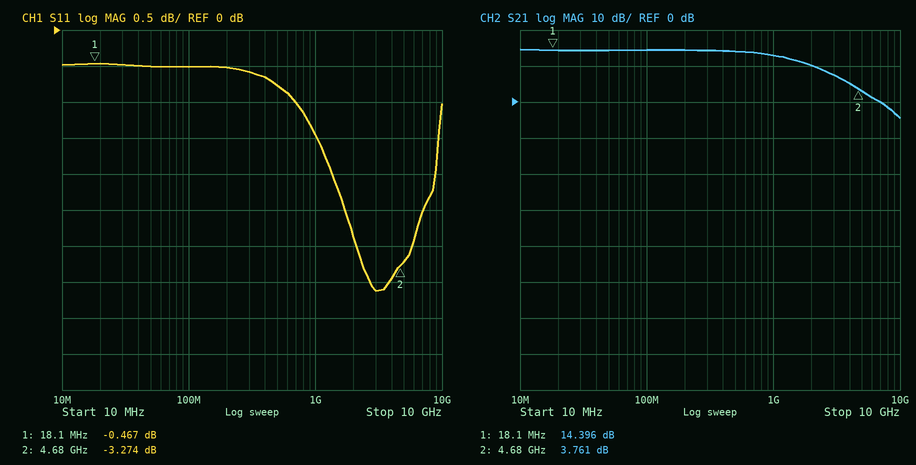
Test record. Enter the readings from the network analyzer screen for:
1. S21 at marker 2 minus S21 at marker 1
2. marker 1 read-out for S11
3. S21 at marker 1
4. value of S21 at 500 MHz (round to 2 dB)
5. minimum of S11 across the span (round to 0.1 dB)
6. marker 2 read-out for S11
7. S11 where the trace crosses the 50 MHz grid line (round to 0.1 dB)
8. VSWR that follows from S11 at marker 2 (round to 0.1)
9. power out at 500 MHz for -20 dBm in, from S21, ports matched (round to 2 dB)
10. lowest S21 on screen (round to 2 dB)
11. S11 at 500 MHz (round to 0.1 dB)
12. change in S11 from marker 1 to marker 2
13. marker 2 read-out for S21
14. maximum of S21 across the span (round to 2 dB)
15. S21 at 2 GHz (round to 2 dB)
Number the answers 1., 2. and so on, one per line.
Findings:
1. -10.635 dB
2. -0.467 dB
3. 14.396 dB
4. 14 dB
5. -3.6 dB
6. -3.274 dB
7. -0.5 dB
8. 5.4
9. -6 dBm
10. -4 dB
11. -0.8 dB
12. -2.807 dB
13. 3.761 dB
14. 14 dB
15. 10 dB
